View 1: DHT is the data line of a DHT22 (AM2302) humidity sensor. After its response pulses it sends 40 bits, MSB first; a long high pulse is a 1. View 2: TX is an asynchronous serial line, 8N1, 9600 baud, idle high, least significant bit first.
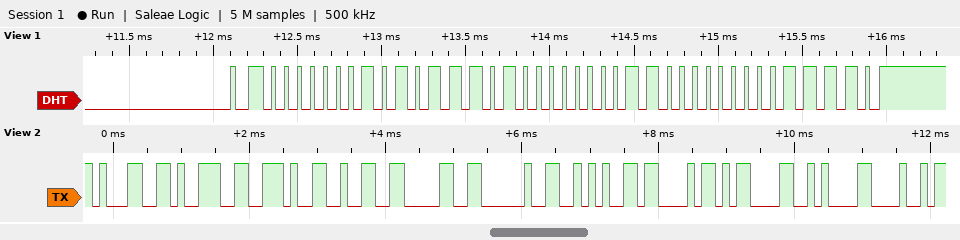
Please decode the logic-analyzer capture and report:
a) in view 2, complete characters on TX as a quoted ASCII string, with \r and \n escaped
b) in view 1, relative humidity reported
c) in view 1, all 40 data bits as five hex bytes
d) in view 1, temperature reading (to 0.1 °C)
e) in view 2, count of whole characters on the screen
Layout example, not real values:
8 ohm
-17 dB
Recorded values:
"19.20 *C\r\nH"
34.9 %
01 5D 00 C0 1E
19.2 °C
11
